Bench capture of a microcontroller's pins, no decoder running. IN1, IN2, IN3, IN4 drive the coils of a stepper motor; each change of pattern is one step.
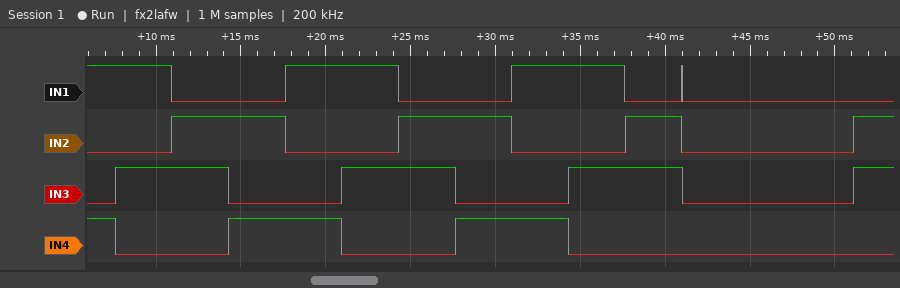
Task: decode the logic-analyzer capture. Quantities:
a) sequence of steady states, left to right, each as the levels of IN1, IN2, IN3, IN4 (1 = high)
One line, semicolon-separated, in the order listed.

1001 1010 0110 0101 1001 1010 0110 0101 1001 1010 0110 0000 0110
